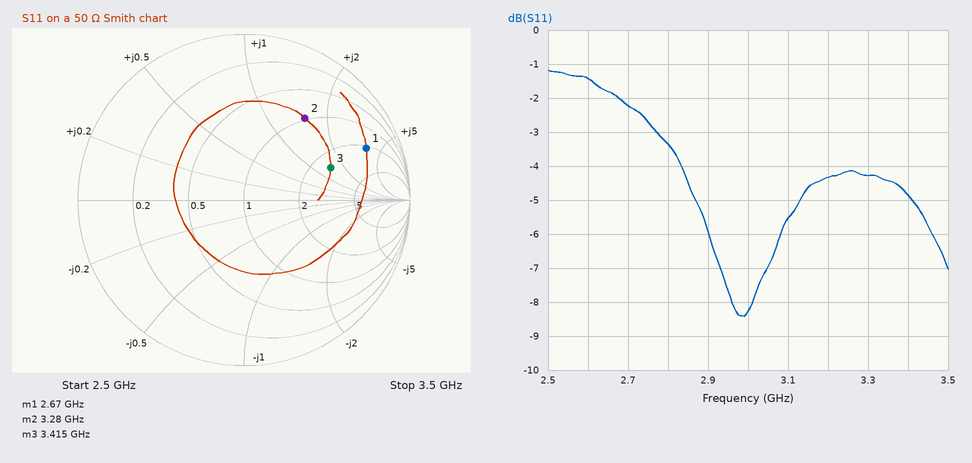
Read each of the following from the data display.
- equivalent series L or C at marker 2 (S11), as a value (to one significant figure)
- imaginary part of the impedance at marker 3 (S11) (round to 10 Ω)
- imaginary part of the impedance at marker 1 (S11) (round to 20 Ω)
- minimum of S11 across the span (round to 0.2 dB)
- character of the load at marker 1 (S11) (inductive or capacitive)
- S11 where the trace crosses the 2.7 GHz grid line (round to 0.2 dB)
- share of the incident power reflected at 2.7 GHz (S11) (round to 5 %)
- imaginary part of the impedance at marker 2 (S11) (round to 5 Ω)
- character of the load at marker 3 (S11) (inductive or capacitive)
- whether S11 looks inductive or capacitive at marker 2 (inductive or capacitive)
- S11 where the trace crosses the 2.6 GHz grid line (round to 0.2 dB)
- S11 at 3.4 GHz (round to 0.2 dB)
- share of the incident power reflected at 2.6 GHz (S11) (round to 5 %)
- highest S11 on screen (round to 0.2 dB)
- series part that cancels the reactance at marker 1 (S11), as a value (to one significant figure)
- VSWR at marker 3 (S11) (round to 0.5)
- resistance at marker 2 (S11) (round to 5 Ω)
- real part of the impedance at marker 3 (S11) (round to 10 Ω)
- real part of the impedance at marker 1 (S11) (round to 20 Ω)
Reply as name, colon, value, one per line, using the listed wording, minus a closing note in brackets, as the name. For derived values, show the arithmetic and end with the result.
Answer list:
equivalent series L or C at marker 2 (S11), as a value: L = 75 Ω/(2π × 3.28 GHz) ≈ 4 nH
imaginary part of the impedance at marker 3 (S11): +70 Ω
imaginary part of the impedance at marker 1 (S11): +180 Ω
minimum of S11 across the span: -8.4 dB
character of the load at marker 1 (S11): inductive
S11 where the trace crosses the 2.7 GHz grid line: -2.2 dB
share of the incident power reflected at 2.7 GHz (S11): 10^(-2.2/10) ≈ 60 %
imaginary part of the impedance at marker 2 (S11): +75 Ω
character of the load at marker 3 (S11): inductive
whether S11 looks inductive or capacitive at marker 2: inductive
S11 where the trace crosses the 2.6 GHz grid line: -1.4 dB
S11 at 3.4 GHz: -4.8 dB
share of the incident power reflected at 2.6 GHz (S11): 10^(-1.4/10) ≈ 72.4 %, so 70 % to the nearest 5 %
highest S11 on screen: -1.2 dB
series part that cancels the reactance at marker 1 (S11), as a value: C = 1/(2π × 2.67 GHz × 180 Ω) ≈ 331 fF, so 300 fF to one significant figure
VSWR at marker 3 (S11): 3.5
resistance at marker 2 (S11): 50 Ω
real part of the impedance at marker 3 (S11): 130 Ω
real part of the impedance at marker 1 (S11): 100 Ω
